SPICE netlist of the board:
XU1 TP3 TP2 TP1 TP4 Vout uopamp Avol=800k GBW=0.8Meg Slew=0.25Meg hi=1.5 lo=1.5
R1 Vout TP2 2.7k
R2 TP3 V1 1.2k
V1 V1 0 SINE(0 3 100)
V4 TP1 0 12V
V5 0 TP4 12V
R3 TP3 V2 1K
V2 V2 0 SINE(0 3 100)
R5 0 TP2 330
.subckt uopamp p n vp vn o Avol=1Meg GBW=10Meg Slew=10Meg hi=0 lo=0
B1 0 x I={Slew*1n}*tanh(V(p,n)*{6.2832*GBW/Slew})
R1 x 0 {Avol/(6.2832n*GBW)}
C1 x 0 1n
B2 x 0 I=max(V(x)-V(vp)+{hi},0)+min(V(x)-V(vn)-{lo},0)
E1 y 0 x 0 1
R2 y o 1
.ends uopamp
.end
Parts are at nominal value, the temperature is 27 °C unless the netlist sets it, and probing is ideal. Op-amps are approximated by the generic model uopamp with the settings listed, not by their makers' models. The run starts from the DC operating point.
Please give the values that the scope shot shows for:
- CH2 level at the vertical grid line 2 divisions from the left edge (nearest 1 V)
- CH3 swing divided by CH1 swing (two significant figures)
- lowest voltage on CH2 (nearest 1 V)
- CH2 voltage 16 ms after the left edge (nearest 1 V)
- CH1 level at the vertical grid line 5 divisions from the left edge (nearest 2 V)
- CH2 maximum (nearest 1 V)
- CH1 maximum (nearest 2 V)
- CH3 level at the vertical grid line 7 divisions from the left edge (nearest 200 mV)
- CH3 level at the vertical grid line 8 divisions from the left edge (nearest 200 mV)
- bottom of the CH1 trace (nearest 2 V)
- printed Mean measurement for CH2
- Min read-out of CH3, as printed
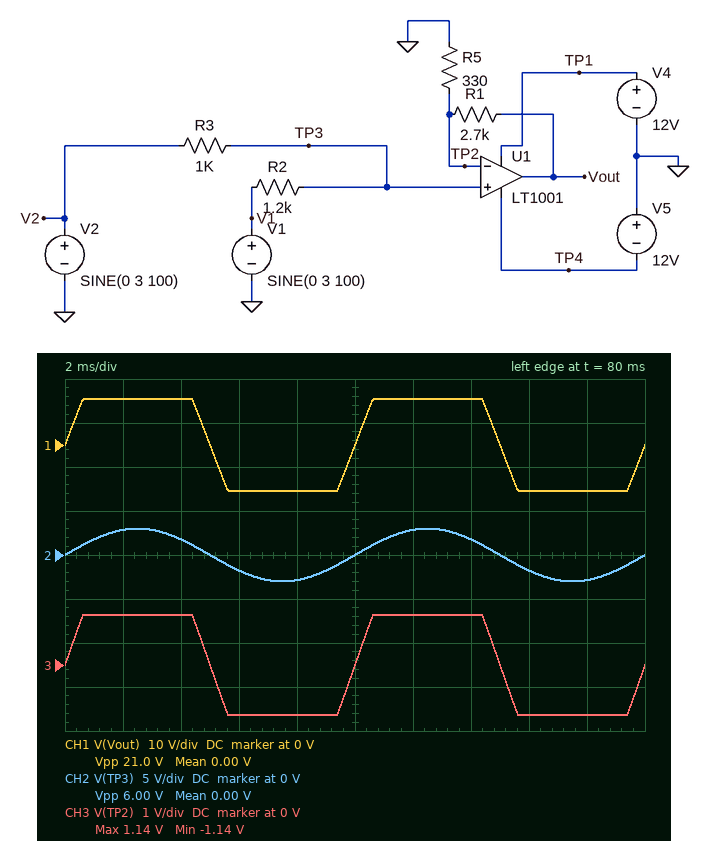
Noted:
2 V
0.11
-3 V
-2 V
0 V
3 V
10 V
1.2 V
-1.2 V
-10 V
0.00 V
-1.14 V
